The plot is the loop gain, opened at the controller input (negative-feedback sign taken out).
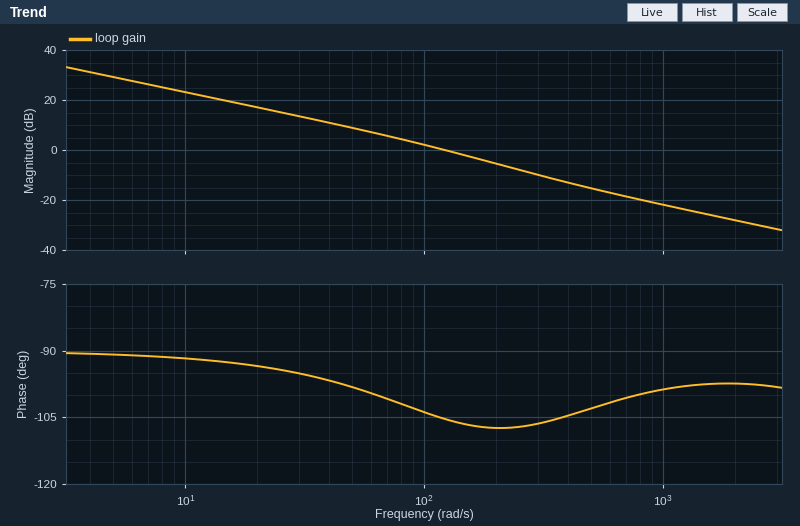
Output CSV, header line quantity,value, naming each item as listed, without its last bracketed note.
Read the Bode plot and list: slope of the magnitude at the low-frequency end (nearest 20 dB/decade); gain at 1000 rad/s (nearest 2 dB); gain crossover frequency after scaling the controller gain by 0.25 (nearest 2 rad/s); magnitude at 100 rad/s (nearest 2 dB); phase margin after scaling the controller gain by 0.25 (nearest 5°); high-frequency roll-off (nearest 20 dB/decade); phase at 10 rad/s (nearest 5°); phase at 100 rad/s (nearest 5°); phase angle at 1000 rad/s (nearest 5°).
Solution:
quantity,value
slope of the magnitude at the low-frequency end,-20 dB/decade
gain at 1000 rad/s,-22 dB
gain crossover frequency after scaling the controller gain by 0.25,36 rad/s
magnitude at 100 rad/s,2 dB
phase margin after scaling the controller gain by 0.25,85°
high-frequency roll-off,-20 dB/decade
phase at 10 rad/s,-90°
phase at 100 rad/s,-105°
phase angle at 1000 rad/s,-100°
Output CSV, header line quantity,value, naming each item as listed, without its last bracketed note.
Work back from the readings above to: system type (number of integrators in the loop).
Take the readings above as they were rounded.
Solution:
quantity,value
system type,1
